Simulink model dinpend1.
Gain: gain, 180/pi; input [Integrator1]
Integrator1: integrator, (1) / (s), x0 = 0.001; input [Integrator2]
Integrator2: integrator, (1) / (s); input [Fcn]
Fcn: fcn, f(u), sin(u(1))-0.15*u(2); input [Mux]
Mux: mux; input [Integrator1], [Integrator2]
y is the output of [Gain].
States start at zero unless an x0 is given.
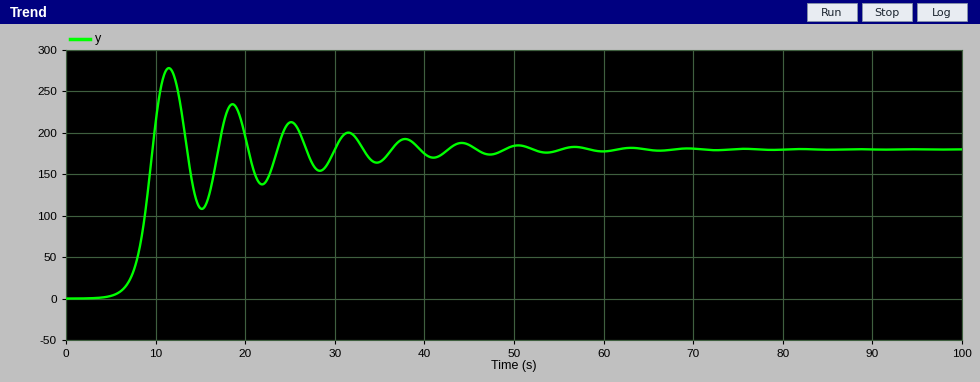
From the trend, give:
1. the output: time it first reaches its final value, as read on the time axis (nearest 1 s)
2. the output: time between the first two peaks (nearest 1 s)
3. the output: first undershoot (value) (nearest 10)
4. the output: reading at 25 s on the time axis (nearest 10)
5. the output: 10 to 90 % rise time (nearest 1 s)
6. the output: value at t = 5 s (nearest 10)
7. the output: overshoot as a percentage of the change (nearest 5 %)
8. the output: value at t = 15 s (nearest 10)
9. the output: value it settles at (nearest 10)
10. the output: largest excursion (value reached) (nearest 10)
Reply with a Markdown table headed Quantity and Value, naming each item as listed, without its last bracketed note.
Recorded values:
| Quantity | Value |
|---|---|
| the output: time it first reaches its final value, as read on the time axis | 10 s |
| the output: time between the first two peaks | 7 s |
| the output: first undershoot (value) | 110 |
| the output: reading at 25 s on the time axis | 210 |
| the output: 10 to 90 % rise time | 3 s |
| the output: value at t = 5 s | 0 |
| the output: overshoot as a percentage of the change | 55 % |
| the output: value at t = 15 s | 110 |
| the output: value it settles at | 180 |
| the output: largest excursion (value reached) | 280 |
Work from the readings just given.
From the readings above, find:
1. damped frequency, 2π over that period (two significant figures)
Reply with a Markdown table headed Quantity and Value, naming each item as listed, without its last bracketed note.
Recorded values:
| Quantity | Value |
|---|---|
| damped frequency, 2π over that period | 0.90 rad/s |
